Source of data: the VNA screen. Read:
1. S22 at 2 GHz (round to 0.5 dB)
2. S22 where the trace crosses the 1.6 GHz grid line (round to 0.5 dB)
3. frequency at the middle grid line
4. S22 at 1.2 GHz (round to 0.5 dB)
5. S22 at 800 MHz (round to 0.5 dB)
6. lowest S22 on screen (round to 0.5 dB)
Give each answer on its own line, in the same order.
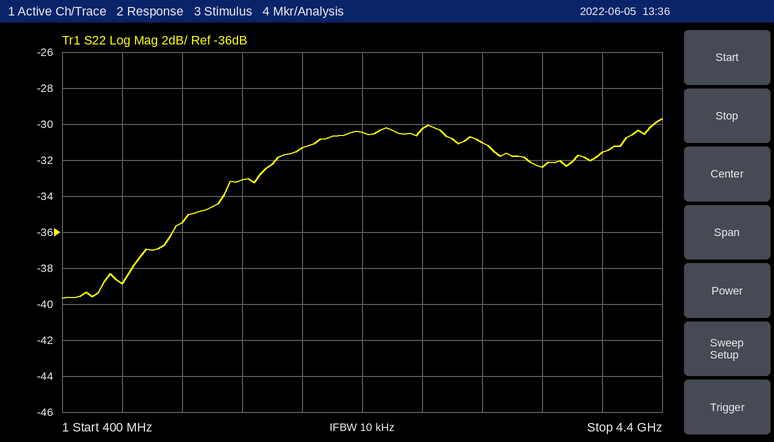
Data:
-31.5 dB
-33.0 dB
2.4 GHz
-35.5 dB
-39.0 dB
-39.5 dB
